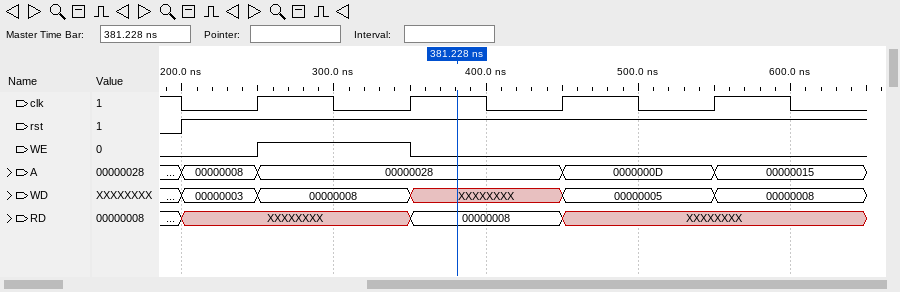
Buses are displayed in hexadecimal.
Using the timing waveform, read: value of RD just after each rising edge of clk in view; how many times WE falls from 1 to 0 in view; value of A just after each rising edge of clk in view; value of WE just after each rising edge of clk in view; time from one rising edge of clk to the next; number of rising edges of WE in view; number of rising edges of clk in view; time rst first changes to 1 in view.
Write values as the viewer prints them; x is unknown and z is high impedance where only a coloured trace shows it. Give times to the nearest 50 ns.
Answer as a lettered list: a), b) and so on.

a) XXXXXXXX, 00000008, XXXXXXXX, XXXXXXXX
b) 1
c) 00000028, 00000028, 0000000D, 00000015
d) 1 0 0 0
e) 100 ns
f) 1
g) 4
h) 200 ns
